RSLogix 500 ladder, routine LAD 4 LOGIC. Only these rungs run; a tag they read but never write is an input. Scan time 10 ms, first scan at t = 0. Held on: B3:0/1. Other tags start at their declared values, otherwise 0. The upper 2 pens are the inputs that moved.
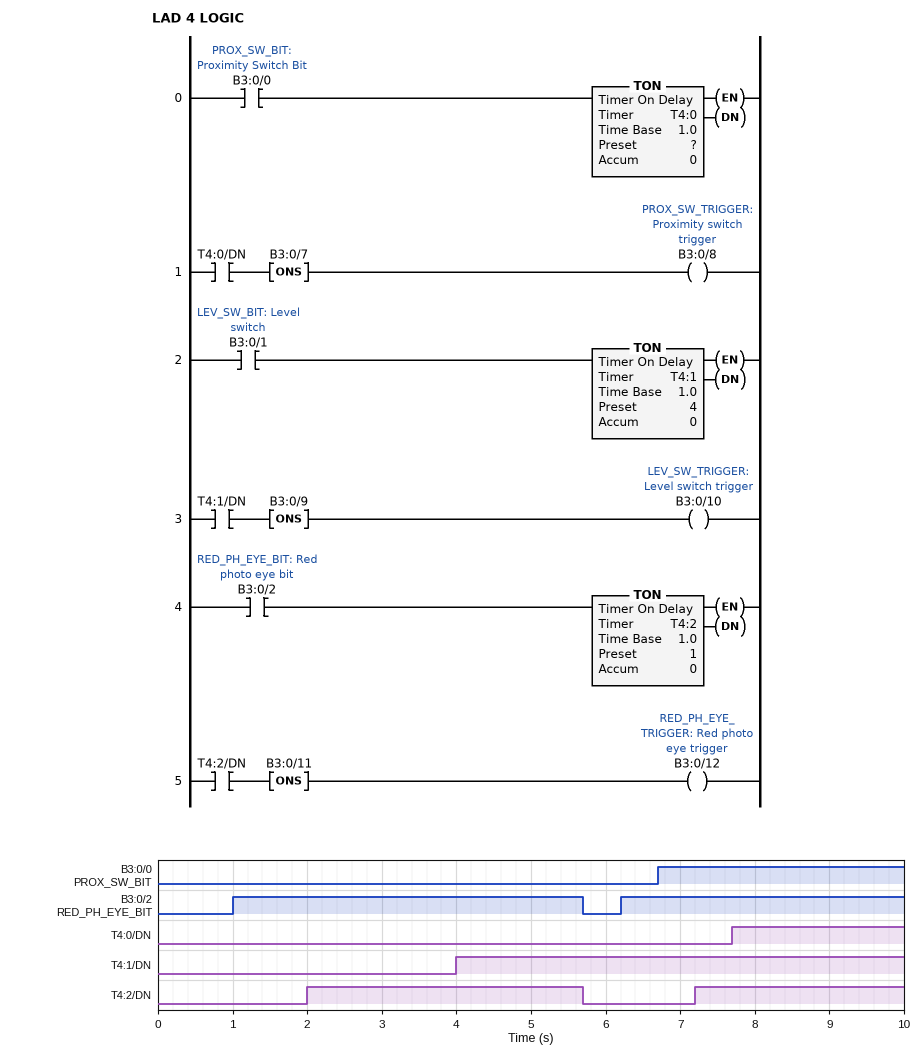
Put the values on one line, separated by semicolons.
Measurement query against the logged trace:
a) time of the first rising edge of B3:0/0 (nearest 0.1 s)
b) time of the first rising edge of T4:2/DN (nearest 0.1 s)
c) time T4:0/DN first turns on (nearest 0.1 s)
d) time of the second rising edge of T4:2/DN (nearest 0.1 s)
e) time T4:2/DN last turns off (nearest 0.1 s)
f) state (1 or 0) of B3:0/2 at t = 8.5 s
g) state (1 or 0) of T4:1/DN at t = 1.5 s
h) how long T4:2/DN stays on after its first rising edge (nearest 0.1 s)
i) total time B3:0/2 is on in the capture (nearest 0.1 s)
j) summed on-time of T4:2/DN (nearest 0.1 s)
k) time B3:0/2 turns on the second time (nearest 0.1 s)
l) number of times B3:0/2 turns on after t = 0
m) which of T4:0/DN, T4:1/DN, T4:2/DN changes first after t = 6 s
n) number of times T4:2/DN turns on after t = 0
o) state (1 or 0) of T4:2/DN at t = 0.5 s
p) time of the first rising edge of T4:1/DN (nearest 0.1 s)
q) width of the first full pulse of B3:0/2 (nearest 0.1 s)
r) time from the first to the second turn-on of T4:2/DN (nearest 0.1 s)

6.7 s; 2.0 s; 7.7 s; 7.2 s; 5.7 s; 1; 0; 3.7 s; 8.5 s; 6.5 s; 6.2 s; 2; T4:2/DN; 2; 0; 4.0 s; 4.7 s; 5.2 s
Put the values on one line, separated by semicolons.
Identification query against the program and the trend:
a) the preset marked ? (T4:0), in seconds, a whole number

1 s
